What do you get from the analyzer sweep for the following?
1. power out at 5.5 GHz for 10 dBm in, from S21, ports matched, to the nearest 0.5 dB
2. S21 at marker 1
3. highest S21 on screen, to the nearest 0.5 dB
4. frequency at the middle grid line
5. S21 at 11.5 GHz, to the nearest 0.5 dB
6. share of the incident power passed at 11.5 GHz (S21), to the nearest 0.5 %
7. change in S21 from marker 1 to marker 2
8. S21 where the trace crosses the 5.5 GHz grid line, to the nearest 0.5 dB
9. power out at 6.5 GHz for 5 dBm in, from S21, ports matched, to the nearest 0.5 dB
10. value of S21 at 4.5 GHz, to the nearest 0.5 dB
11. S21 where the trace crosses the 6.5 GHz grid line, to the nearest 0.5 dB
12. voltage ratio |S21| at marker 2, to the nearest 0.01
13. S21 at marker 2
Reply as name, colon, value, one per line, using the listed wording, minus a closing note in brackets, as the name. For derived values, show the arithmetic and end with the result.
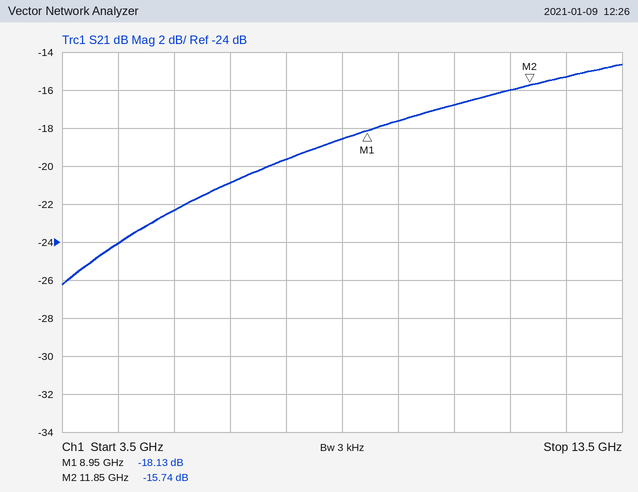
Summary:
power out at 5.5 GHz for 10 dBm in, from S21, ports matched, to the nearest 0.5 dB: 10 dBm + (-22.5 dB) = -12.5 dBm
S21 at marker 1: -18.13 dB
highest S21 on screen, to the nearest 0.5 dB: -14.5 dB
frequency at the middle grid line: 8.5 GHz
S21 at 11.5 GHz, to the nearest 0.5 dB: -16.0 dB
share of the incident power passed at 11.5 GHz (S21), to the nearest 0.5 %: 10^(-16/10) ≈ 2.5 %
change in S21 from marker 1 to marker 2: -15.74 − (-18.13) = 2.39 dB
S21 where the trace crosses the 5.5 GHz grid line, to the nearest 0.5 dB: -22.5 dB
power out at 6.5 GHz for 5 dBm in, from S21, ports matched, to the nearest 0.5 dB: 5 dBm + (-21.0 dB) = -16.0 dBm
value of S21 at 4.5 GHz, to the nearest 0.5 dB: -24.0 dB
S21 where the trace crosses the 6.5 GHz grid line, to the nearest 0.5 dB: -21.0 dB
voltage ratio |S21| at marker 2, to the nearest 0.01: 10^(-15.74/20) ≈ 0.16
S21 at marker 2: -15.74 dB
